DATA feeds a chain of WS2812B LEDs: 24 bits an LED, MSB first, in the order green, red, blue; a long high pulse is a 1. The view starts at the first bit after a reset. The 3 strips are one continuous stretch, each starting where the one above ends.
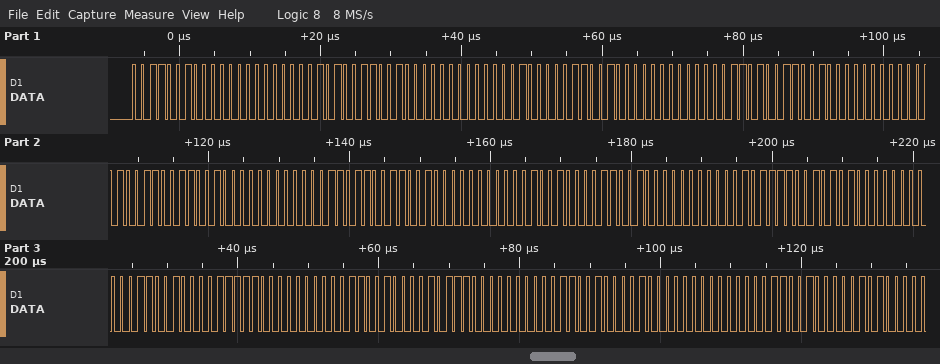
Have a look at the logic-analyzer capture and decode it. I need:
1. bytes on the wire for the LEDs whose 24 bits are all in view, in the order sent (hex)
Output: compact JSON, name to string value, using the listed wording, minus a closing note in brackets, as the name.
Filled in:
{"bytes on the wire for the LEDs whose 24 bits are all in view, in the order sent": "32 00 05 32 00 08 32 00 0D 32 00 13 32 00 1B 32 00 24 32 00 2F 2A 00 32 1F 00 32 17 00 32 10 00 32"}
